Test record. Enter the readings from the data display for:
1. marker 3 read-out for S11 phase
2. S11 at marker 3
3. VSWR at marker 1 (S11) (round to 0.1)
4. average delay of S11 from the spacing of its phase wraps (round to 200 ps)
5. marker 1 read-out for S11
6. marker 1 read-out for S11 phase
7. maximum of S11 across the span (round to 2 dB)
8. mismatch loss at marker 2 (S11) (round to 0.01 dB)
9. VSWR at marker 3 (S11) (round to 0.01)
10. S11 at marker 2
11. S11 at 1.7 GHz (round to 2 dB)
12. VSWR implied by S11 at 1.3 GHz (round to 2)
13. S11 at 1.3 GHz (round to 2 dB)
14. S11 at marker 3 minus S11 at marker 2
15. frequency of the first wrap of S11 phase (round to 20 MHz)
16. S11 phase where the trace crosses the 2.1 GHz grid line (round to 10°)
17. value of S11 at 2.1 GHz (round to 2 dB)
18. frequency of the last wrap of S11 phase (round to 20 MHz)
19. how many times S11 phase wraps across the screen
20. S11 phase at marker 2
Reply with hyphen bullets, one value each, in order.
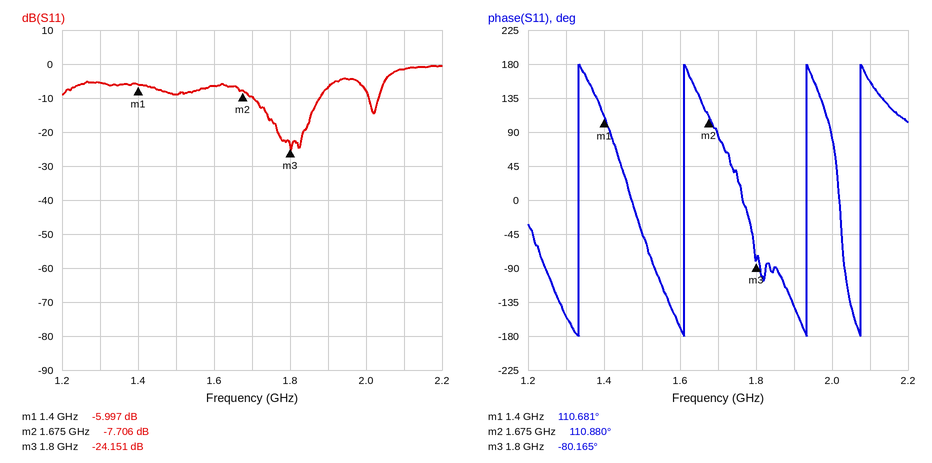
- -80.165°
- -24.151 dB
- 3.0
- 4.0 ns
- -5.997 dB
- 110.681°
- 0 dB
- 0.81 dB
- 1.13
- -7.706 dB
- -10 dB
- 4
- -6 dB
- -16.445 dB
- 1.34 GHz
- 160°
- -2 dB
- 2.08 GHz
- 4
- 110.880°
